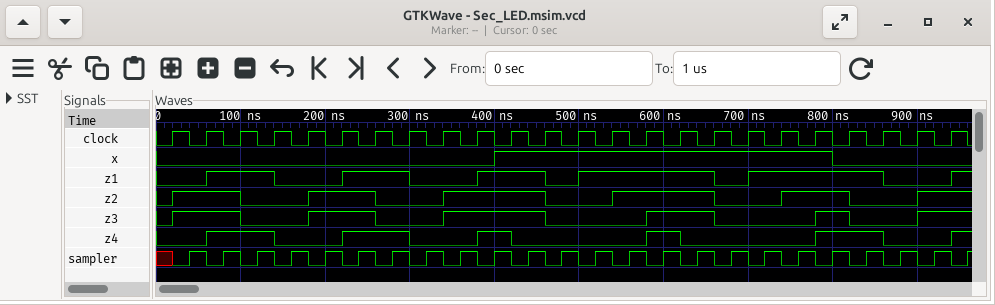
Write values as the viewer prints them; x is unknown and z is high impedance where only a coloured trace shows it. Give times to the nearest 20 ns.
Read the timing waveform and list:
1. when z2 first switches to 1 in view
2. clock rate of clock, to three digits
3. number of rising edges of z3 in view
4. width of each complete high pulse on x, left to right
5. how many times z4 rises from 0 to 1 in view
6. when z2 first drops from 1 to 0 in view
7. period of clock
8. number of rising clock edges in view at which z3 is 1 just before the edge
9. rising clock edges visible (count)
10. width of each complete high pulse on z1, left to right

20 ns
25.0 MHz
6
400 ns
6
100 ns
40 ns
11
24
80 ns, 80 ns, 80 ns, 160 ns, 160 ns
